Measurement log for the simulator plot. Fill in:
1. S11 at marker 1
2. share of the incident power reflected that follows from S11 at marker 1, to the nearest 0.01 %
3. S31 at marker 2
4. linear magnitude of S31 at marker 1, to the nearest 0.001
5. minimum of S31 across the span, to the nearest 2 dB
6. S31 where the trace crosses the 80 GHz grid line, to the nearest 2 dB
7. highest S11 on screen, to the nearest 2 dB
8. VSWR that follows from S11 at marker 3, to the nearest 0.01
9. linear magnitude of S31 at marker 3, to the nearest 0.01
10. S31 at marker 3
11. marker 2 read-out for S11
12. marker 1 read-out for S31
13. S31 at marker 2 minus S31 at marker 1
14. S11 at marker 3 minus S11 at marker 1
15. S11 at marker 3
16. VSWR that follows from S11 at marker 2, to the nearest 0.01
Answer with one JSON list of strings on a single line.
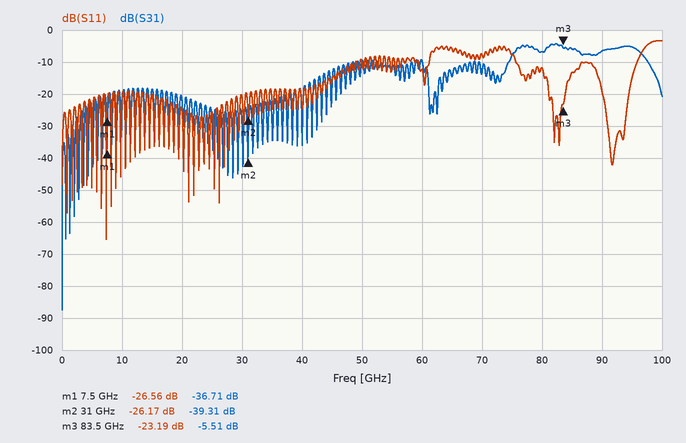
["-26.56 dB", "0.22 %", "-39.31 dB", "0.015", "-88 dB", "-6 dB", "-4 dB", "1.15", "0.53", "-5.51 dB", "-26.17 dB", "-36.71 dB", "-2.60 dB", "3.37 dB", "-23.19 dB", "1.10"]
